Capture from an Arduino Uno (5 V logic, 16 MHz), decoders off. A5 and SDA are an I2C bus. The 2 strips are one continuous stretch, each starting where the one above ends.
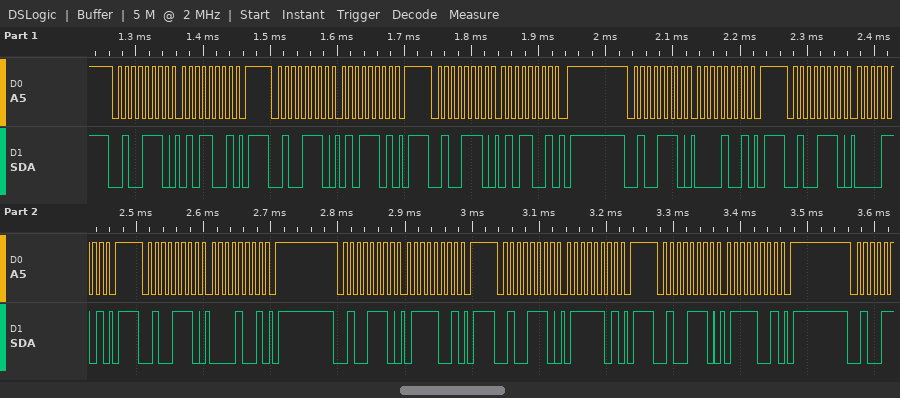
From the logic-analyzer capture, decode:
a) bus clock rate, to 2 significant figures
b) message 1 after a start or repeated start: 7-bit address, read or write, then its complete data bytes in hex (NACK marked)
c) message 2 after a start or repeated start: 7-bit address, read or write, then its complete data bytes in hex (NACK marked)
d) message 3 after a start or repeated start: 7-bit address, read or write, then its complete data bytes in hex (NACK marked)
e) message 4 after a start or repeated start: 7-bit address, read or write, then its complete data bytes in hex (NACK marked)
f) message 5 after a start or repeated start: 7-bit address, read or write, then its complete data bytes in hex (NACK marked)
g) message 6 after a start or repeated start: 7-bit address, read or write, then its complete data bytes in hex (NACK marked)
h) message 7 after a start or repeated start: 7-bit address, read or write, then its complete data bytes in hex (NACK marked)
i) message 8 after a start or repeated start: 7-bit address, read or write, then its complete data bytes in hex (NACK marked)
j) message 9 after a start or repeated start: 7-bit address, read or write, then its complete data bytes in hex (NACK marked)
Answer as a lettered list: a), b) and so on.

a) 100 kHz
b) 0x27 write: 59
c) 0x27 write: 5D
d) 0x27 write: 59
e) 0x27 write: 09
f) 0x27 write: 0D
g) 0x27 write: 09
h) 0x27 write: 79
i) 0x27 write: 7D
j) 0x27 write: 79
